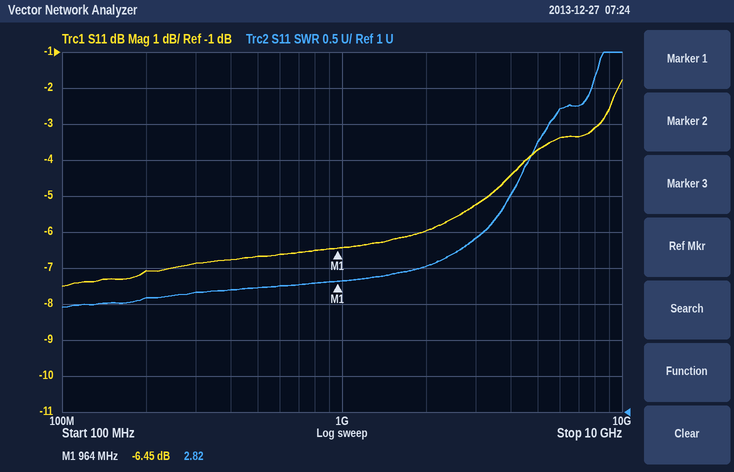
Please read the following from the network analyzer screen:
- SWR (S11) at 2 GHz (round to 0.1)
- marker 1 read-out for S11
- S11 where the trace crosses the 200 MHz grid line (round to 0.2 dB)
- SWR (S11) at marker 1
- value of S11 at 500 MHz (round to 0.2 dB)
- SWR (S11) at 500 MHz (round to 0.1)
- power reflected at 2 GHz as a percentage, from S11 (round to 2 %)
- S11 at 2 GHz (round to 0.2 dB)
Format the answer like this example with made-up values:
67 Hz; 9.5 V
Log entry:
3.0; -6.45 dB; -7.0 dB; 2.82; -6.6 dB; 2.7; 26 %; -6.0 dB
